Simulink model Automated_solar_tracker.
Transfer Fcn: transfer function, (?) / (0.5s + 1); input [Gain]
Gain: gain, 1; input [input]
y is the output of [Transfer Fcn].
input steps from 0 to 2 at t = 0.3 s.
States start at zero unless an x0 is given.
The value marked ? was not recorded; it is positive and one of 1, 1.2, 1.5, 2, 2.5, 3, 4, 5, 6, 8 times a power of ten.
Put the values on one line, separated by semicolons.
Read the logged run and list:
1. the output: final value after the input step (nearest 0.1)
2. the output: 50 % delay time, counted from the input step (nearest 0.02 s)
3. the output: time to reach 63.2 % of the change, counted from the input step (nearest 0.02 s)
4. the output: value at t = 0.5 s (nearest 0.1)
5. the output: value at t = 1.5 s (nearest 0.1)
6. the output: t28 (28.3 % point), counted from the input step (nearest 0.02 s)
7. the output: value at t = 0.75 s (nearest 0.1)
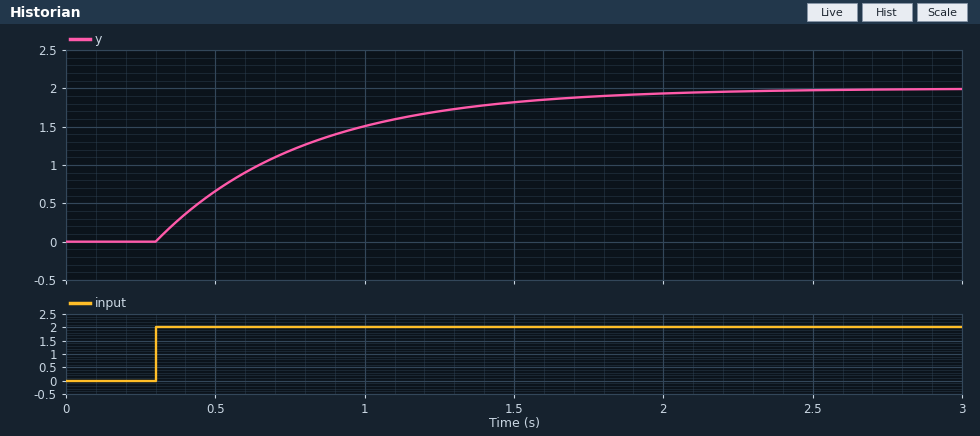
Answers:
2.0; 0.34 s; 0.50 s; 0.7; 1.8; 0.16 s; 1.2
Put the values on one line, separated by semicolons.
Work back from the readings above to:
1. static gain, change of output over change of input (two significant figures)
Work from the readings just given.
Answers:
1.0
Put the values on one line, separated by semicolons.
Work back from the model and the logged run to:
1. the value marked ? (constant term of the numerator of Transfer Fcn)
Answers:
1
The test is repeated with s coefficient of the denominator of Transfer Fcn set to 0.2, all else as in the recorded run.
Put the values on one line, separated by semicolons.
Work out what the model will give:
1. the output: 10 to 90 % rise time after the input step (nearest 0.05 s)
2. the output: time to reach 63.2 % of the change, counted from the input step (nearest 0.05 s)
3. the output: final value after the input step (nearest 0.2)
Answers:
0.45 s; 0.20 s; 2.0
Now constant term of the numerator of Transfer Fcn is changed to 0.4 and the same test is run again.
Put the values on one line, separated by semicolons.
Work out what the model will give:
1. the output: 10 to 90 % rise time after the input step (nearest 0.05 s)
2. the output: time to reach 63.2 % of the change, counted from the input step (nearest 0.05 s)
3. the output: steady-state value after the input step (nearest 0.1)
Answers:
1.10 s; 0.50 s; 0.8
